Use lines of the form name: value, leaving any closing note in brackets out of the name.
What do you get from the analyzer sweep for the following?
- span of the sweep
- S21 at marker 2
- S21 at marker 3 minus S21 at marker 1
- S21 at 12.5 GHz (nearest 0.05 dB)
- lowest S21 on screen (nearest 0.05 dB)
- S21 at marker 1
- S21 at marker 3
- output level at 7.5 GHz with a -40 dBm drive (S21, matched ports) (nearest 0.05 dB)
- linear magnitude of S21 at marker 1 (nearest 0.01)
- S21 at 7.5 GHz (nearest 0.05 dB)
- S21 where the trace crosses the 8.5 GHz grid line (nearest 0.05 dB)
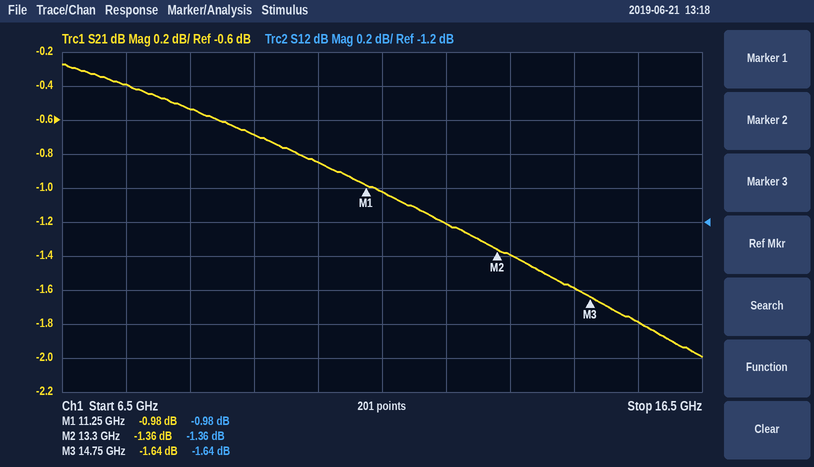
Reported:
span of the sweep: 10 GHz
S21 at marker 2: -1.36 dB
S21 at marker 3 minus S21 at marker 1: -0.66 dB
S21 at 12.5 GHz: -1.20 dB
lowest S21 on screen: -2.00 dB
S21 at marker 1: -0.98 dB
S21 at marker 3: -1.64 dB
output level at 7.5 GHz with a -40 dBm drive (S21, matched ports): -40.40 dBm
linear magnitude of S21 at marker 1: 0.89
S21 at 7.5 GHz: -0.40 dB
S21 where the trace crosses the 8.5 GHz grid line: -0.55 dB
